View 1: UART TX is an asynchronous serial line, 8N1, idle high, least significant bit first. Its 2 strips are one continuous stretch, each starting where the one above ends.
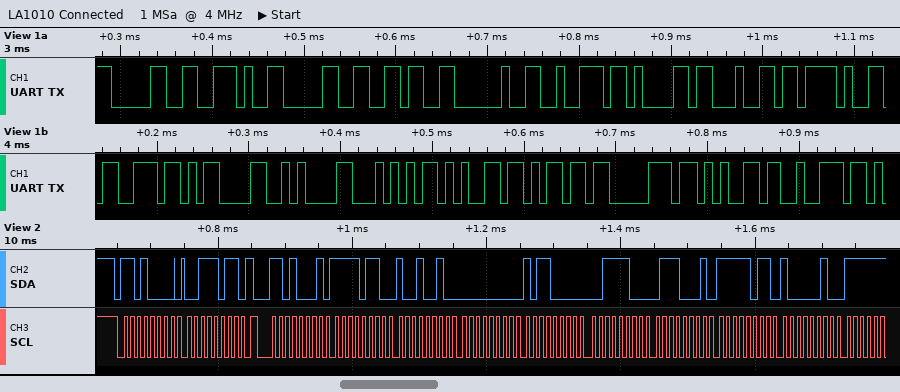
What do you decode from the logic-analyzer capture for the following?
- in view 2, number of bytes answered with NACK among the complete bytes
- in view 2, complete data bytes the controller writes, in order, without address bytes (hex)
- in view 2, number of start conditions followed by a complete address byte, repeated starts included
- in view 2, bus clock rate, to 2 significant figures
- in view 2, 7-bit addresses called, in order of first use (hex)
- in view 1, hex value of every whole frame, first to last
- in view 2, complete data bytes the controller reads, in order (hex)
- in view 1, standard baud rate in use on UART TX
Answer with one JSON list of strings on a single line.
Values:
["0", "3B", "2", "100 kHz", "0x68", "0x30 0x2E 0x30 0x36 0x20 0x72 0x61 0x64 0x2F 0x73 0x0D 0x0A 0x54 0x65 0x6D 0x70 0x65 0x72", "F6 92 00 B0 3C 71 FB 82", "115200 baud"]
